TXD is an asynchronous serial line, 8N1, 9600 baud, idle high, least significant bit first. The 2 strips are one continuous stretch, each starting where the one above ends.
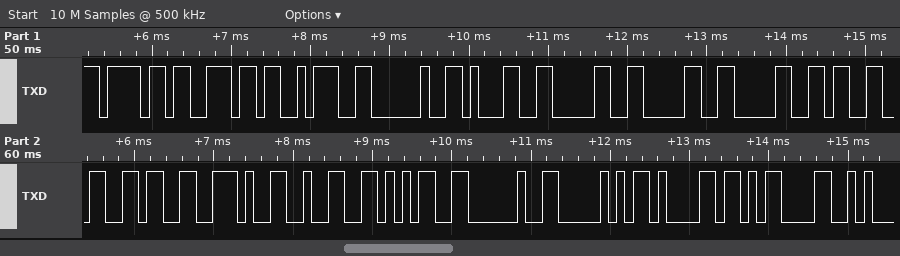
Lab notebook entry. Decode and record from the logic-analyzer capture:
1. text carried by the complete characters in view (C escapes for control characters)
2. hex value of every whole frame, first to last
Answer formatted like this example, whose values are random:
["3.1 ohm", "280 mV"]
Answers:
["\"on: 100036.25 Pa\\r\"", "0x6F 0x6E 0x3A 0x20 0x31 0x30 0x30 0x30 0x33 0x36 0x2E 0x32 0x35 0x20 0x50 0x61 0x0D"]
